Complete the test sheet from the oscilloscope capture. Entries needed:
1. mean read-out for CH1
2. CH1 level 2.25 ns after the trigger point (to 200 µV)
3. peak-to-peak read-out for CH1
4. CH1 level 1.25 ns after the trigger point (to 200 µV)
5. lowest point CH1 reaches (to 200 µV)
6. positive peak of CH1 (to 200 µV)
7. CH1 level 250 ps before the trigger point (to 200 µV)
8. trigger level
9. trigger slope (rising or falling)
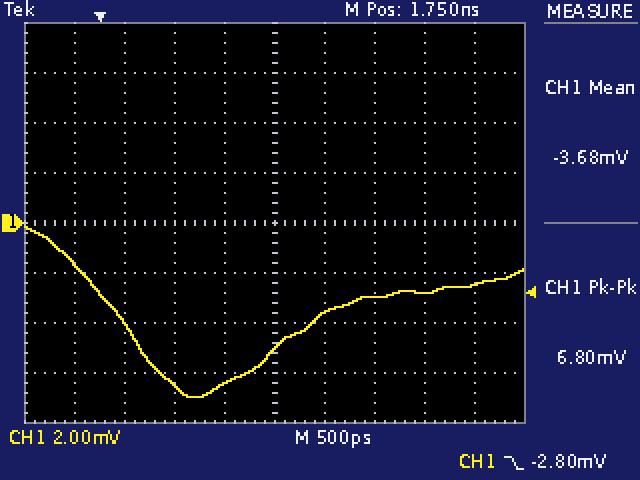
-3.68 mV
-3.6 mV
6.80 mV
-6.4 mV
-7.0 mV
-200 µV
-1.6 mV
-2.80 mV
falling
